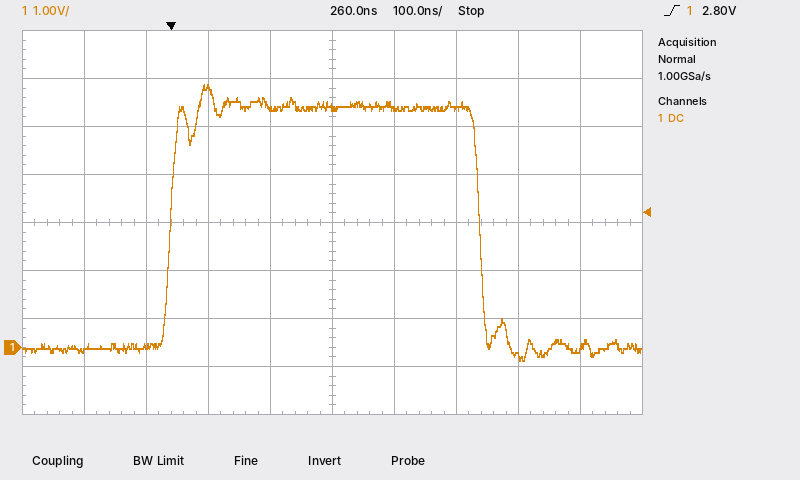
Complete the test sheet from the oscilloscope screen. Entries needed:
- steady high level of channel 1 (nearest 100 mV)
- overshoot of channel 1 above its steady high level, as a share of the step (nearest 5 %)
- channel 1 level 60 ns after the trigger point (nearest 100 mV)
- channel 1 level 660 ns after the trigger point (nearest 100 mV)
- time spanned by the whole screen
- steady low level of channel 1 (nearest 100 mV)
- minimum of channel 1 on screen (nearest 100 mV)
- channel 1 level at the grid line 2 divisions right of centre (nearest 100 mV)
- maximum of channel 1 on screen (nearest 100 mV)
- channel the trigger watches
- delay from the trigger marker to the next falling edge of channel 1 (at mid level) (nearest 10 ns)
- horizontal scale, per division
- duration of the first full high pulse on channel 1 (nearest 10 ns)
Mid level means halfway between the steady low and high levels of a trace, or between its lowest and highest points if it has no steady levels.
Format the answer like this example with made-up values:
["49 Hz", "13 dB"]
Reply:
["5.0 V", "10 %", "5.4 V", "0.0 V", "1 µs", "0.0 V", "-300 mV", "5.0 V", "5.5 V", "channel 1", "500 ns", "100 ns", "500 ns"]
